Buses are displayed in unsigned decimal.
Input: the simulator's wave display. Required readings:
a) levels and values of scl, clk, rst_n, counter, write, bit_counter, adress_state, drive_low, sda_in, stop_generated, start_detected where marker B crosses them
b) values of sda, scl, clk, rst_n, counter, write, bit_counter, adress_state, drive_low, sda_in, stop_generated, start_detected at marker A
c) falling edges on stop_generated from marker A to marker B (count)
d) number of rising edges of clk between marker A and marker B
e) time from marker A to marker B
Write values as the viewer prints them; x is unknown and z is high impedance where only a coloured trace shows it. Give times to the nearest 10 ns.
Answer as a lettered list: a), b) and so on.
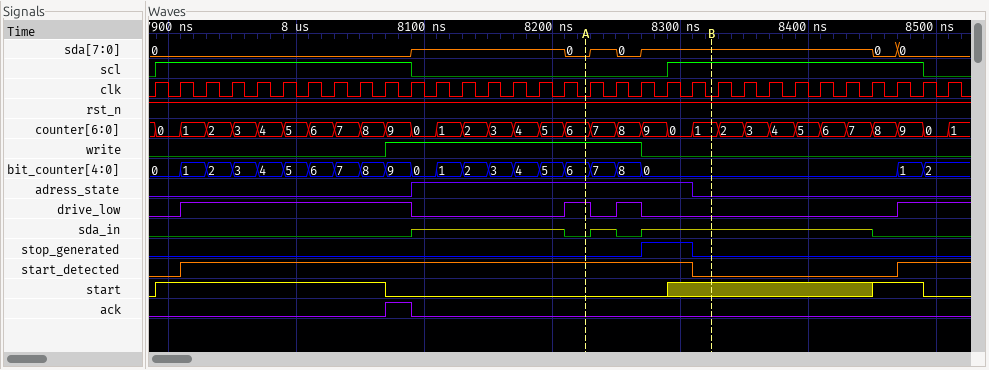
a) scl=1, clk=0, rst_n=1, counter=1, write=0, bit_counter=0, adress_state=0, drive_low=0, sda_in=z, stop_generated=0, start_detected=0
b) sda=0, scl=0, clk=0, rst_n=1, counter=6, write=1, bit_counter=6, adress_state=1, drive_low=1, sda_in=0, stop_generated=0, start_detected=1
c) 1
d) 5
e) 100 ns
